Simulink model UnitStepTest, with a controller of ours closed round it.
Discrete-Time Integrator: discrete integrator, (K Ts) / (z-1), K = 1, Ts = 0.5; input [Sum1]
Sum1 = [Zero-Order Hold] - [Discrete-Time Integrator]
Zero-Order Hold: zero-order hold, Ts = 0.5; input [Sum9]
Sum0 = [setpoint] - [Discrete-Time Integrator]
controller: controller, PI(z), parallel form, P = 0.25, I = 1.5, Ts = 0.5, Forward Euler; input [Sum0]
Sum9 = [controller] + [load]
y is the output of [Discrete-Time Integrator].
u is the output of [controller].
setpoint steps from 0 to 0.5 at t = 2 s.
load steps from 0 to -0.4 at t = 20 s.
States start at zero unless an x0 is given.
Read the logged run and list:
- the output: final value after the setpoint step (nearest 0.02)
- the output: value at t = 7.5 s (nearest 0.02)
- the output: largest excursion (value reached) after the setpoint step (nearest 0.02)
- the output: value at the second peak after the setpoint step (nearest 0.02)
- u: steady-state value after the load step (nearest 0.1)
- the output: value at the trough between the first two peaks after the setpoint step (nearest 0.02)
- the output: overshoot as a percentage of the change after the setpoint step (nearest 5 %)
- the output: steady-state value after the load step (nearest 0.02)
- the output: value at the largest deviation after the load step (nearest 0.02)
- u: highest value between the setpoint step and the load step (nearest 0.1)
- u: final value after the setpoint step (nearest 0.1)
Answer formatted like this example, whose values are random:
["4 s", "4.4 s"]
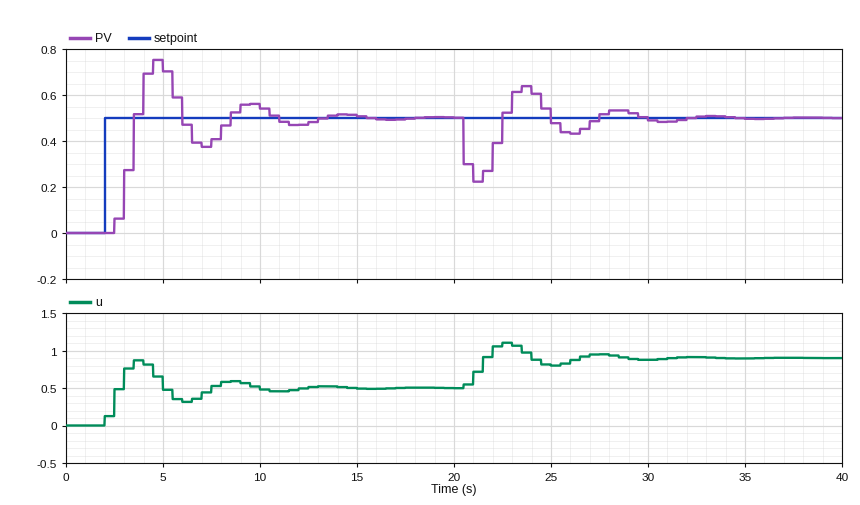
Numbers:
["0.50", "0.40", "0.76", "0.56", "0.9", "0.38", "50 %", "0.50", "0.22", "0.9", "0.5"]
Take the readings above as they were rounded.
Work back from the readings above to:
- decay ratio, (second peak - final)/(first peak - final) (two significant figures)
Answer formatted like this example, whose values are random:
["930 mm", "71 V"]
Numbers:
["0.23"]
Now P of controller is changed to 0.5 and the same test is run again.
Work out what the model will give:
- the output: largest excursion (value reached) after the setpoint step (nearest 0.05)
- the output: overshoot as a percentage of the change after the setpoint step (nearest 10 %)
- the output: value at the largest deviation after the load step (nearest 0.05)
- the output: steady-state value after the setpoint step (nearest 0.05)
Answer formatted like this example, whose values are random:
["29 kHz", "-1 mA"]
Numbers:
["0.65", "30 %", "0.25", "0.50"]
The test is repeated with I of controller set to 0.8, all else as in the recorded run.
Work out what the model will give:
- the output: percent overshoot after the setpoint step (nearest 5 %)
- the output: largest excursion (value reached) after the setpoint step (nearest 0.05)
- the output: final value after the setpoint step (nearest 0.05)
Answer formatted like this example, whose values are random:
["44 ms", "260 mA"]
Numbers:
["15 %", "0.55", "0.50"]
